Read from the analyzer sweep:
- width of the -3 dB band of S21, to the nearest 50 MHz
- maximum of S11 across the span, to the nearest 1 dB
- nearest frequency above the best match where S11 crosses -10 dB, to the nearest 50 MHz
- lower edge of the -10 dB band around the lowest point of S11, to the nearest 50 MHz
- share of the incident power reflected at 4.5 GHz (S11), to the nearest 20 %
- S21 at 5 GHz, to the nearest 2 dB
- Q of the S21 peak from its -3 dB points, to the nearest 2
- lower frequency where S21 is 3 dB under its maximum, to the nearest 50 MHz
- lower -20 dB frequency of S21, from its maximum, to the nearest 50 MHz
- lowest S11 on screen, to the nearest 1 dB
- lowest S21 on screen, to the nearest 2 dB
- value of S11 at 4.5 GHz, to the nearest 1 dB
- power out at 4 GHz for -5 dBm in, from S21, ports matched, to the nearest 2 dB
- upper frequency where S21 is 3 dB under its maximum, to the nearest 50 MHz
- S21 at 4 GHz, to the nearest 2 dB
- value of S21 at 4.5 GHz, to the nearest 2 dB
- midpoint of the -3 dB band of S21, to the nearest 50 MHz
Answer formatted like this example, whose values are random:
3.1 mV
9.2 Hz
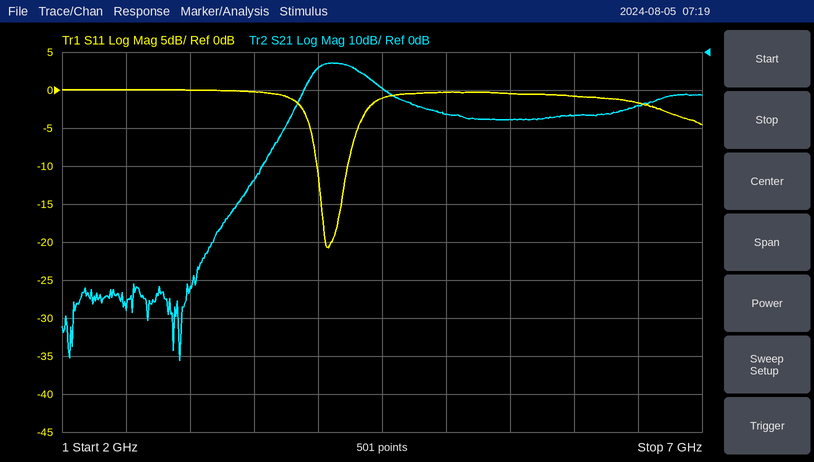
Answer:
400 MHz
0 dB
4.25 GHz
4.00 GHz
80 %
-16 dB
10
3.95 GHz
3.70 GHz
-21 dB
-82 dB
-1 dB
-10 dBm
4.35 GHz
-4 dB
-10 dB
4.15 GHz
